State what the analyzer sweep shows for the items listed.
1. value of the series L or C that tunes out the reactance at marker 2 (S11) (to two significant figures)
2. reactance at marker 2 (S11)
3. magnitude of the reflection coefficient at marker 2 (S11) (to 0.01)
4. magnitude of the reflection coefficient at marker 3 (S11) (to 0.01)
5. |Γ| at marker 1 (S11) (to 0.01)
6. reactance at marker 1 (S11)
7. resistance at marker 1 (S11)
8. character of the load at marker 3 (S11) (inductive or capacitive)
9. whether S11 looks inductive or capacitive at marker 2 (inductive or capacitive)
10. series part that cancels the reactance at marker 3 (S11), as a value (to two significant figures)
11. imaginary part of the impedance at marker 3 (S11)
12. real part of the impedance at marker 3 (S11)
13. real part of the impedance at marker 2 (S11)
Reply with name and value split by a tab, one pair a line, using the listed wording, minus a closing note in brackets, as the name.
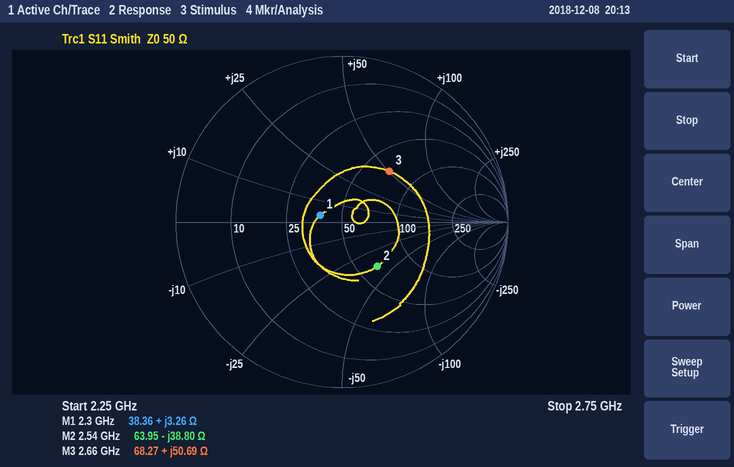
value of the series L or C that tunes out the reactance at marker 2 (S11)	2.4 nH
reactance at marker 2	-38.80 Ω
magnitude of the reflection coefficient at marker 2 (S11)	0.34
magnitude of the reflection coefficient at marker 3 (S11)	0.42
|Γ| at marker 1 (S11)	0.14
reactance at marker 1	+3.26 Ω
resistance at marker 1	38.36 Ω
character of the load at marker 3 (S11)	inductive
whether S11 looks inductive or capacitive at marker 2	capacitive
series part that cancels the reactance at marker 3 (S11), as a value	1.2 pF
imaginary part of the impedance at marker 3	+50.69 Ω
real part of the impedance at marker 3	68.27 Ω
real part of the impedance at marker 2	63.95 Ω
